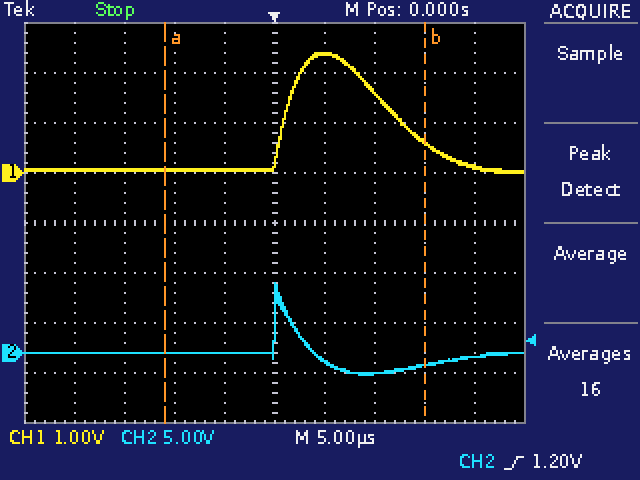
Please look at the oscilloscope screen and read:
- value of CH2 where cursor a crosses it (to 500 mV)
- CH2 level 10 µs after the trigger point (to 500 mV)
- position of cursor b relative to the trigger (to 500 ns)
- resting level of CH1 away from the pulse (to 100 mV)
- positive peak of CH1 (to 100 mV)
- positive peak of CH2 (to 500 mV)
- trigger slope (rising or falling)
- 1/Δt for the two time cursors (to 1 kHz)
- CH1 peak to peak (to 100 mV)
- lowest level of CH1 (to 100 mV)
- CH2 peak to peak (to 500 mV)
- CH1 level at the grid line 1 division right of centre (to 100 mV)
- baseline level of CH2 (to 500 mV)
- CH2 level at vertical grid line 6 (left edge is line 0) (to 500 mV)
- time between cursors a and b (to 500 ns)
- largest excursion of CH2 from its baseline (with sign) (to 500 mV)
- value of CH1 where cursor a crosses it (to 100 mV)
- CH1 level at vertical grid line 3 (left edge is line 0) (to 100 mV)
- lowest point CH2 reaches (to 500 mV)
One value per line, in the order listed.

0.0 V
-2.0 V
+15.0 µs
100 mV
2.4 V
7.0 V
rising
38 kHz
2.4 V
0.0 V
9.0 V
2.4 V
0.0 V
-1.0 V
26.0 µs
+7.0 V
100 mV
100 mV
-2.0 V
